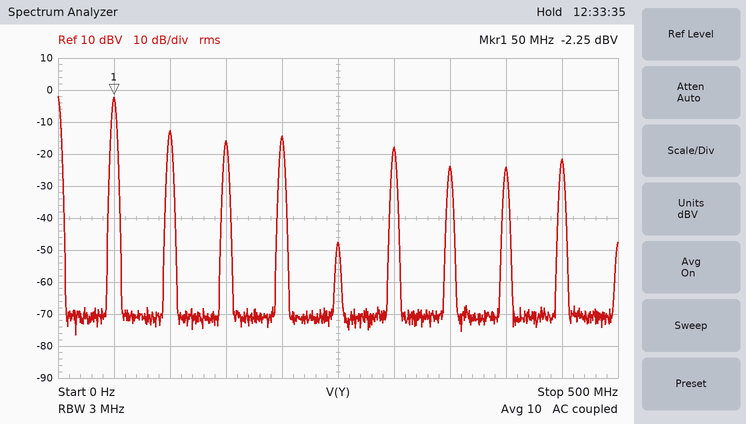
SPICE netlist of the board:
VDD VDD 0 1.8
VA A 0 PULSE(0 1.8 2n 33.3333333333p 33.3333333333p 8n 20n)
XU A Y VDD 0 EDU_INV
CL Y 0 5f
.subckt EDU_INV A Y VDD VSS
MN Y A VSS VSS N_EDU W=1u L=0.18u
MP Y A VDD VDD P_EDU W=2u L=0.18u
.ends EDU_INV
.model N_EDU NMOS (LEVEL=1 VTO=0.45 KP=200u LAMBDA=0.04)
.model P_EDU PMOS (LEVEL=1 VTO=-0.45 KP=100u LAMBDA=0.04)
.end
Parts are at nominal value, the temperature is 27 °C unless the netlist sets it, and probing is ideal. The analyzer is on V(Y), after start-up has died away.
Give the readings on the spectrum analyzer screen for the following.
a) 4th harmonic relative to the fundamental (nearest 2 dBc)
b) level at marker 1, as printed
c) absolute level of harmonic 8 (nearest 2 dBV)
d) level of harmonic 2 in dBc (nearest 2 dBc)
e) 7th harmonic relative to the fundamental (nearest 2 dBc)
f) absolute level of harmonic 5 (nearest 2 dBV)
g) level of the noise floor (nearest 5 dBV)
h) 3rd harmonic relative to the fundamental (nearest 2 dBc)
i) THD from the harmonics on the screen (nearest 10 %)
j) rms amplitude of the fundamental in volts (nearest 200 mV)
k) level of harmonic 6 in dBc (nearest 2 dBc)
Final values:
-12 dBc
-2.25 dBV
-24 dBV
-10 dBc
-22 dBc
-48 dBV
-70 dBV
-14 dBc
50 %
800 mV
-16 dBc
